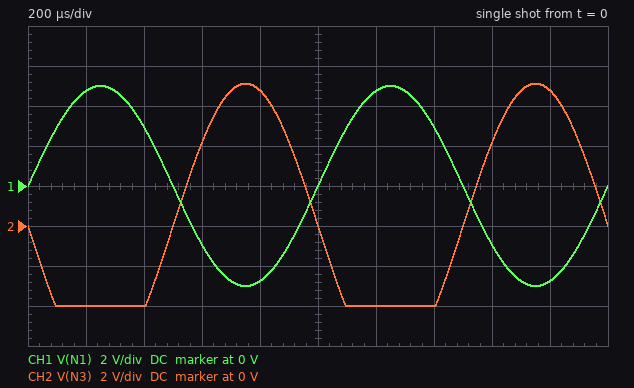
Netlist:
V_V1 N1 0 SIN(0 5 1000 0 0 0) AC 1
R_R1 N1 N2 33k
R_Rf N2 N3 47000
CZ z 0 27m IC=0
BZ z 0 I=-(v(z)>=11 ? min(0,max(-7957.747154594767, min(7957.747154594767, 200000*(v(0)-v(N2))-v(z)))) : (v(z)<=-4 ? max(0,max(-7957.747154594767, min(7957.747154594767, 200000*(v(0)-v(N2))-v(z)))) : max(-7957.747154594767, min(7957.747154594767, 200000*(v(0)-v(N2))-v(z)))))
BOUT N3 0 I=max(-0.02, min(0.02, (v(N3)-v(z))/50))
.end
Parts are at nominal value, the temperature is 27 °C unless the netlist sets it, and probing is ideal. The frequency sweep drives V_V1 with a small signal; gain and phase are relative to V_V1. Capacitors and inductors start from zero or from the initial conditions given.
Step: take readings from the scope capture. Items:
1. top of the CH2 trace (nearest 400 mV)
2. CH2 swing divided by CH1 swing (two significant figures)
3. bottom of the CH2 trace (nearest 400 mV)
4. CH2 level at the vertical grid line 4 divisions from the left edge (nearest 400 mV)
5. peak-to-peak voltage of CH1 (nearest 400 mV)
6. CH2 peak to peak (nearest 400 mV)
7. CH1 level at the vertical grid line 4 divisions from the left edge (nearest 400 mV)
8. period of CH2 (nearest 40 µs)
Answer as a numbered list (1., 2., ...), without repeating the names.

1. 7.2 V
2. 1.1
3. -4.0 V
4. 6.8 V
5. 10.0 V
6. 11.2 V
7. -4.8 V
8. 1.00 ms
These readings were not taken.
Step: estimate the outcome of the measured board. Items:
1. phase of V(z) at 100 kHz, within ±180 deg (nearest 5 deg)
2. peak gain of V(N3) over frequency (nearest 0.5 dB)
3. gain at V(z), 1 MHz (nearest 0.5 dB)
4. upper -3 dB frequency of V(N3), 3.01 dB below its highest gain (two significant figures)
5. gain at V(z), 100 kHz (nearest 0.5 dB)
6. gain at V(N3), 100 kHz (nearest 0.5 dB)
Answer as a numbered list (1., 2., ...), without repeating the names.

1. 170 deg
2. 3.0 dB
3. -4.0 dB
4. 490 kHz
5. 3.0 dB
6. 3.0 dB
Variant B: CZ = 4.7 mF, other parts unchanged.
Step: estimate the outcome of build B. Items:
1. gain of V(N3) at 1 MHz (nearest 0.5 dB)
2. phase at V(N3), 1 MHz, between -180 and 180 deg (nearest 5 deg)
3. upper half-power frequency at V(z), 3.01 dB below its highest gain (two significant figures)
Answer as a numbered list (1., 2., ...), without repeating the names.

1. 2.5 dB
2. 160 deg
3. 2.8 MHz
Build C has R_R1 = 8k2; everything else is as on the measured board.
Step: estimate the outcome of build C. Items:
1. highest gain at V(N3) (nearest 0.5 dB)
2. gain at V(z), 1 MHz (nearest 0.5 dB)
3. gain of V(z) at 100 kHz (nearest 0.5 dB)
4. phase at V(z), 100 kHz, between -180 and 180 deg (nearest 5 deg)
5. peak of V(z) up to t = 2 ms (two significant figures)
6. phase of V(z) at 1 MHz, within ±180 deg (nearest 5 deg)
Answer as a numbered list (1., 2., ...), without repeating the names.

1. 15.0 dB
2. 0 dB
3. 14.0 dB
4. 150 deg
5. 11 V
6. 100 deg
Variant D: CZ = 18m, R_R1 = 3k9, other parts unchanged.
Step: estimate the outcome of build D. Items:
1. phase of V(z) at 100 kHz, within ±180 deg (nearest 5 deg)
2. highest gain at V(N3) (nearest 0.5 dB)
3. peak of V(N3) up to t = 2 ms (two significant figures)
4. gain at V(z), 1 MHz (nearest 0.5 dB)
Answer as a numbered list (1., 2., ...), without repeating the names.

1. 145 deg
2. 21.5 dB
3. 11 V
4. 4.0 dB
